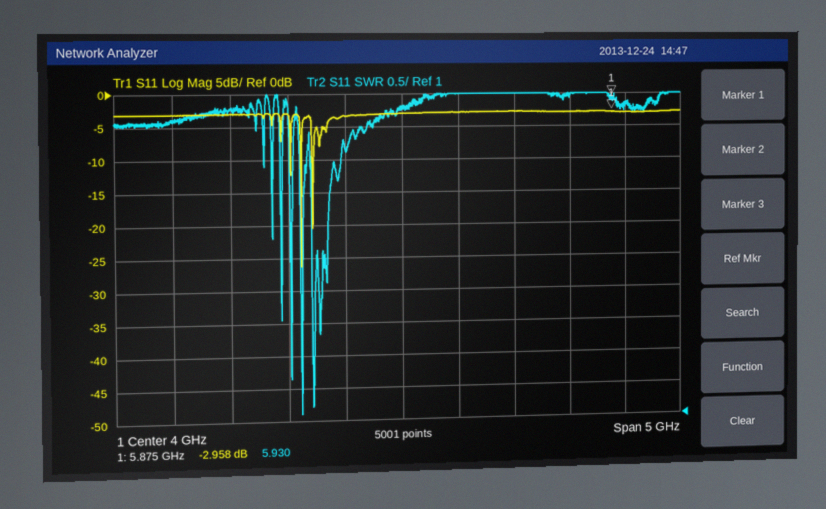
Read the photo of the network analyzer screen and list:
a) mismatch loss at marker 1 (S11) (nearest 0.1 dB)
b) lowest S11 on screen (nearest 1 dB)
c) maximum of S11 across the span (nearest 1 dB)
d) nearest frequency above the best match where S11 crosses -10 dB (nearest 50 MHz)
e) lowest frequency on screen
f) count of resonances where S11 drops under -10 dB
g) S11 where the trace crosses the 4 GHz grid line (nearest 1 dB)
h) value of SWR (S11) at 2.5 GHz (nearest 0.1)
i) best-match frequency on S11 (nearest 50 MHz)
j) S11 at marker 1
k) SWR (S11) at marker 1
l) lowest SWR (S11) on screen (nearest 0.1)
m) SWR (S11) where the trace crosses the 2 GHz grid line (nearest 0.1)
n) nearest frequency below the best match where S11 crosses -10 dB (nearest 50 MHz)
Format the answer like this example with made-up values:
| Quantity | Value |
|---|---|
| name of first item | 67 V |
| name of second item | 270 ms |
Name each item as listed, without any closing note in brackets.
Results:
| Quantity | Value |
|---|---|
| mismatch loss at marker 1 (S11) | 3.1 dB |
| lowest S11 on screen | -26 dB |
| maximum of S11 across the span | -3 dB |
| nearest frequency above the best match where S11 crosses -10 dB | 3.10 GHz |
| lowest frequency on screen | 1.5 GHz |
| count of resonances where S11 drops under -10 dB | 3 |
| S11 where the trace crosses the 4 GHz grid line | -3 dB |
| value of SWR (S11) at 2.5 GHz | 5.8 |
| best-match frequency on S11 | 3.10 GHz |
| S11 at marker 1 | -2.958 dB |
| SWR (S11) at marker 1 | 5.930 |
| lowest SWR (S11) on screen | 1.1 |
| SWR (S11) where the trace crosses the 2 GHz grid line | 5.6 |
| nearest frequency below the best match where S11 crosses -10 dB | 3.10 GHz |
